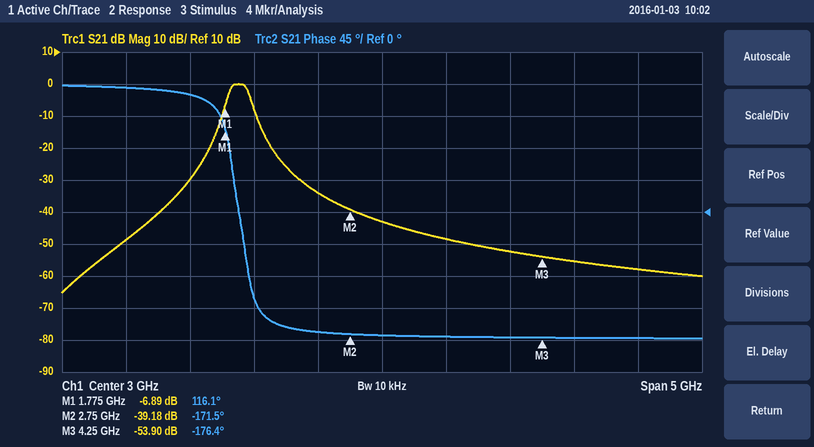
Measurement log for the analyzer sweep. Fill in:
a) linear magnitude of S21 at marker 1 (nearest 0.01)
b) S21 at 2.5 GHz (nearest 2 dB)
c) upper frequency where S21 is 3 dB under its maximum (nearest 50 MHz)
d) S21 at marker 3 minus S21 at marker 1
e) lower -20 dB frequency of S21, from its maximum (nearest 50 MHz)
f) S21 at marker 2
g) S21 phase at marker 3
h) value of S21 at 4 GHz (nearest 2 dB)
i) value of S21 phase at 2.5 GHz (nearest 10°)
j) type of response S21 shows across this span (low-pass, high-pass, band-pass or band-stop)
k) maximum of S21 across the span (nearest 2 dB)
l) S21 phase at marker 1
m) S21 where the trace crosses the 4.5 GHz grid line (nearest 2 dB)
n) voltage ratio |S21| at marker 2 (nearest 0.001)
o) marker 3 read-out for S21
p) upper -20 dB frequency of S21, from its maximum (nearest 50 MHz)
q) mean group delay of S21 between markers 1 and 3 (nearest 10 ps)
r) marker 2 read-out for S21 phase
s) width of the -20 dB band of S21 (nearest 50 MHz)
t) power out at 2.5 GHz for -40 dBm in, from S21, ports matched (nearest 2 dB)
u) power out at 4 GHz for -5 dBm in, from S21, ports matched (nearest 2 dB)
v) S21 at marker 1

0.45
-34 dB
1.95 GHz
-47.01 dB
1.65 GHz
-39.18 dB
-176.4°
-52 dB
-170°
band-pass
0 dB
116.1°
-56 dB
0.011
-53.90 dB
2.15 GHz
330 ps
-171.5°
500 MHz
-74 dBm
-58 dBm
-6.89 dB
